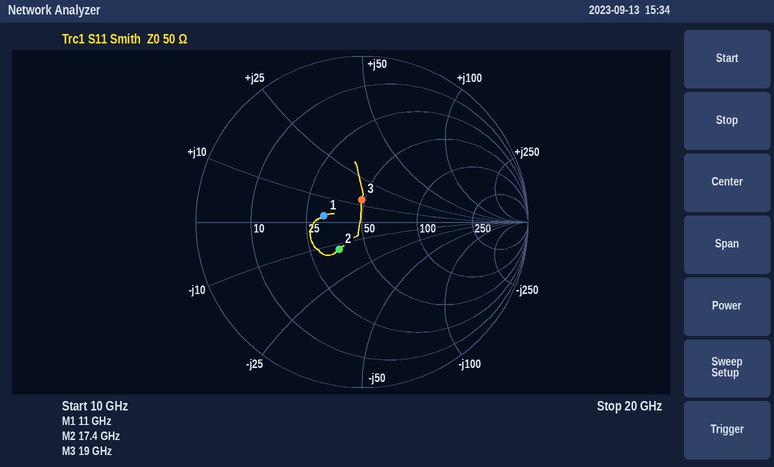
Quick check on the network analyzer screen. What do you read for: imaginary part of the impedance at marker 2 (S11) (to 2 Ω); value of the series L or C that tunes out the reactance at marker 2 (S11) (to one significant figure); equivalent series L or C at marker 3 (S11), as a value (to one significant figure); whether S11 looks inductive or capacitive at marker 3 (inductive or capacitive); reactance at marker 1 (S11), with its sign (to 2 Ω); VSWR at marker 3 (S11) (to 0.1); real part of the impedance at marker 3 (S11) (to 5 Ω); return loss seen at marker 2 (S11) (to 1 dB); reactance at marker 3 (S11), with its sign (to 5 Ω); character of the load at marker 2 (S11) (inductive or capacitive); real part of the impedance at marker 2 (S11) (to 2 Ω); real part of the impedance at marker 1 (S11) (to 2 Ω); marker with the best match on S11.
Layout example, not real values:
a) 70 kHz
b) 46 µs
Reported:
a) -12 Ω
b) 100 pH
c) 100 pH
d) inductive
e) +2 Ω
f) 1.3
g) 50 Ω
h) 13 dB
i) +15 Ω
j) capacitive
k) 36 Ω
l) 32 Ω
m) marker 3
